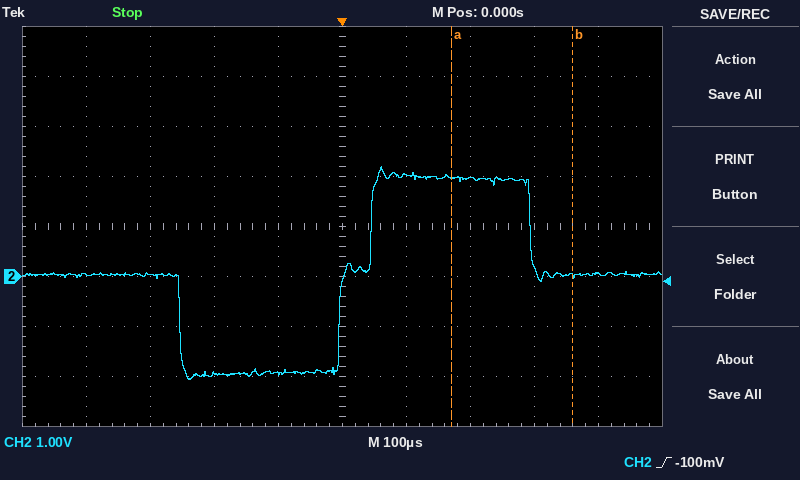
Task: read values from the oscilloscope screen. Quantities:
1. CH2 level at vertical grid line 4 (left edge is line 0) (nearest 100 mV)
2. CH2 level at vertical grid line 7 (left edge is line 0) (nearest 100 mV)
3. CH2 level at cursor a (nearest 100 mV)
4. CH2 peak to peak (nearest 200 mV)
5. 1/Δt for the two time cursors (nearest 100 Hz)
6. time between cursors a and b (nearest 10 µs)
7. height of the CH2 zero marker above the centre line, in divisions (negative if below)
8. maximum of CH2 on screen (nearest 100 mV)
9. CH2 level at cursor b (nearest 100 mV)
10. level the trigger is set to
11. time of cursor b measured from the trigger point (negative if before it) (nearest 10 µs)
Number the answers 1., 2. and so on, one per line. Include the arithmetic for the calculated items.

1. -1.9 V
2. 2.0 V
3. 2.0 V
4. 4.2 V
5. 1 / 190 µs ≈ 5.3 kHz
6. 190 µs
7. -1.0 div
8. 2.2 V
9. 0.0 V
10. -100 mV
11. +360 µs
